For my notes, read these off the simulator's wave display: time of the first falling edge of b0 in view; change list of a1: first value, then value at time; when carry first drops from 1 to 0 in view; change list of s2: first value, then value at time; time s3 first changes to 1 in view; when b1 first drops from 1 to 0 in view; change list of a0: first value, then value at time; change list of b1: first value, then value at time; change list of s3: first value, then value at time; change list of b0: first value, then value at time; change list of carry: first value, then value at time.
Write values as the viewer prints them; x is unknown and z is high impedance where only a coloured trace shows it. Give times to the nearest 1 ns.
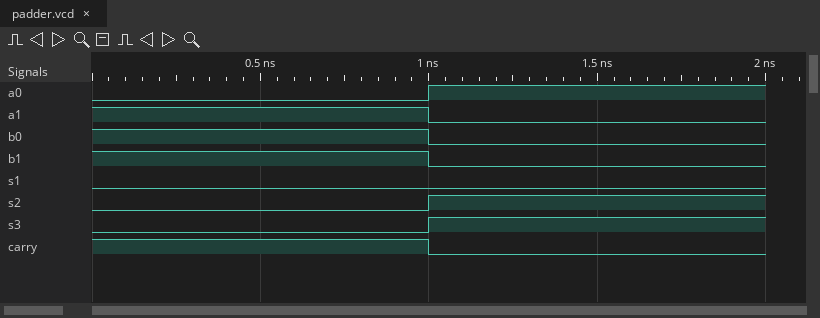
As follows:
1 ns
1, 0 at 1 ns
1 ns
0, 1 at 1 ns
1 ns
1 ns
0, 1 at 1 ns
1, 0 at 1 ns
0, 1 at 1 ns
1, 0 at 1 ns
1, 0 at 1 ns
